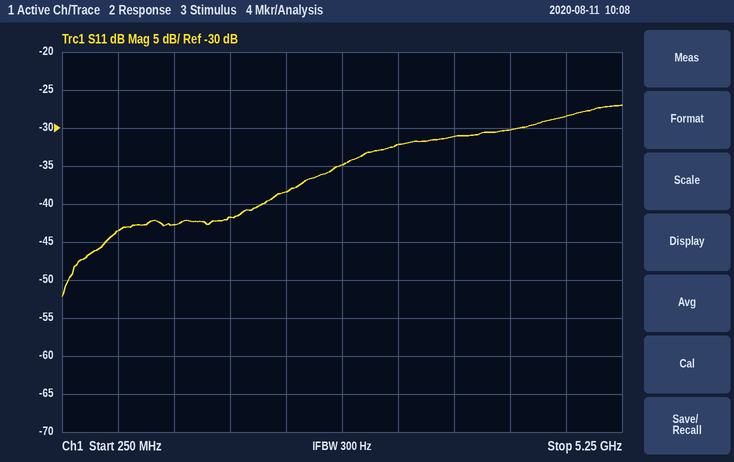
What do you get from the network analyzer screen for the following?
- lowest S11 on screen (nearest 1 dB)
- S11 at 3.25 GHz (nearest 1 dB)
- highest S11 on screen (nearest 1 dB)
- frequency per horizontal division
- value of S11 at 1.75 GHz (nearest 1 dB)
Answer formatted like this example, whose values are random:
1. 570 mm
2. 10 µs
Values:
1. -52 dB
2. -32 dB
3. -27 dB
4. 500 MHz
5. -42 dB
